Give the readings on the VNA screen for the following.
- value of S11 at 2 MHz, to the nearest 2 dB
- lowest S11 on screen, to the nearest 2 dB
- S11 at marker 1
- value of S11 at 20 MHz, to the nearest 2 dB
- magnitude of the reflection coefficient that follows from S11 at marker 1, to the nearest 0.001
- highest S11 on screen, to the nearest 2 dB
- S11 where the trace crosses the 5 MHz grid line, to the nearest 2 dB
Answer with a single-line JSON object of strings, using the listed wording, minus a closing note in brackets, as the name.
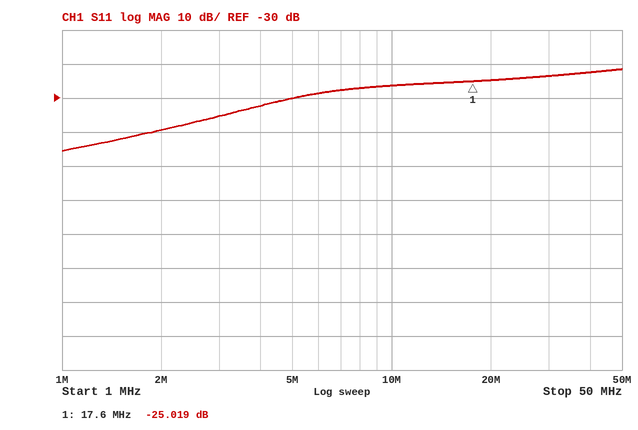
{"value of S11 at 2 MHz, to the nearest 2 dB": "-40 dB", "lowest S11 on screen, to the nearest 2 dB": "-46 dB", "S11 at marker 1": "-25.019 dB", "value of S11 at 20 MHz, to the nearest 2 dB": "-24 dB", "magnitude of the reflection coefficient that follows from S11 at marker 1, to the nearest 0.001": "0.056", "highest S11 on screen, to the nearest 2 dB": "-22 dB", "S11 where the trace crosses the 5 MHz grid line, to the nearest 2 dB": "-30 dB"}
